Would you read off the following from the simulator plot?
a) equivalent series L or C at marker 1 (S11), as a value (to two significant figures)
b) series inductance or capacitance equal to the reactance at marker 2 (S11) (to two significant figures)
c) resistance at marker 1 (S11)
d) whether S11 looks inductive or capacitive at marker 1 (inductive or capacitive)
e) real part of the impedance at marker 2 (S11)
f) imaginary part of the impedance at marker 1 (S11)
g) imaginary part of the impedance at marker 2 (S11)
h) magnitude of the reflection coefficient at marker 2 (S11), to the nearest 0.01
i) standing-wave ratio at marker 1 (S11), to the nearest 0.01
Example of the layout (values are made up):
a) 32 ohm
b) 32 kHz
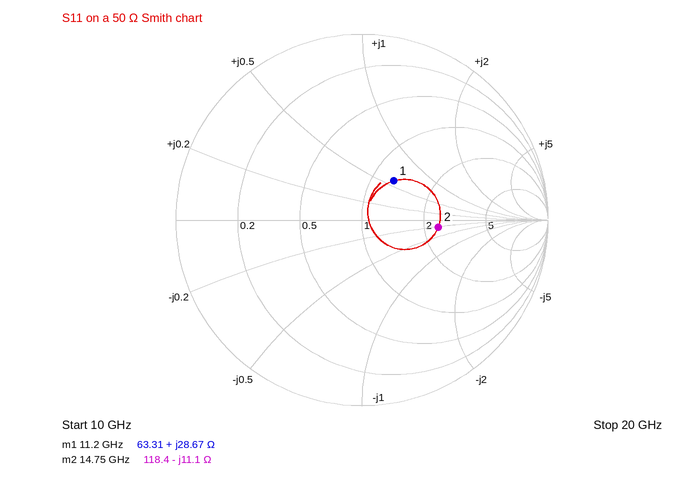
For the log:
a) 410 pH
b) 970 fF
c) 63.31 Ω
d) inductive
e) 118.4 Ω
f) +28.67 Ω
g) -11.1 Ω
h) 0.41
i) 1.74
